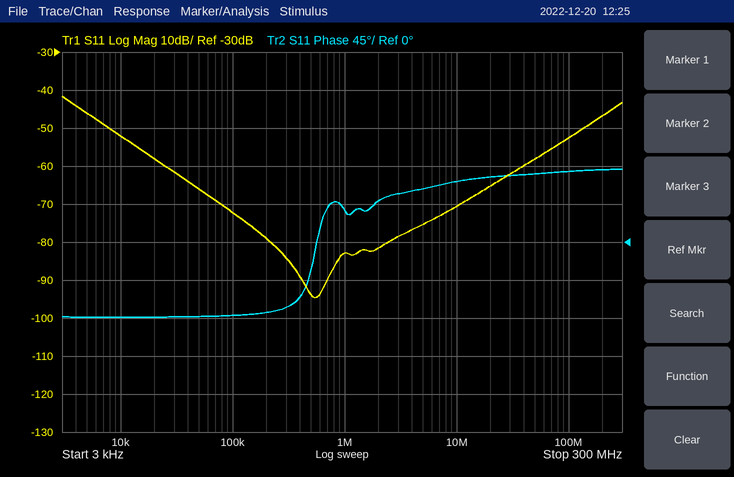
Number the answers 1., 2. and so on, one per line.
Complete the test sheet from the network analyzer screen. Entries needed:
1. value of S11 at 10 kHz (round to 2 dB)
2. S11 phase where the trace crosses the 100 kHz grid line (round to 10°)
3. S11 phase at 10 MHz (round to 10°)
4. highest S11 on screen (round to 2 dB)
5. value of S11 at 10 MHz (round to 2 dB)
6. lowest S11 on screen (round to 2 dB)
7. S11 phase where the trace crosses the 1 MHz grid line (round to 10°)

1. -52 dB
2. -90°
3. 70°
4. -42 dB
5. -70 dB
6. -94 dB
7. 40°
